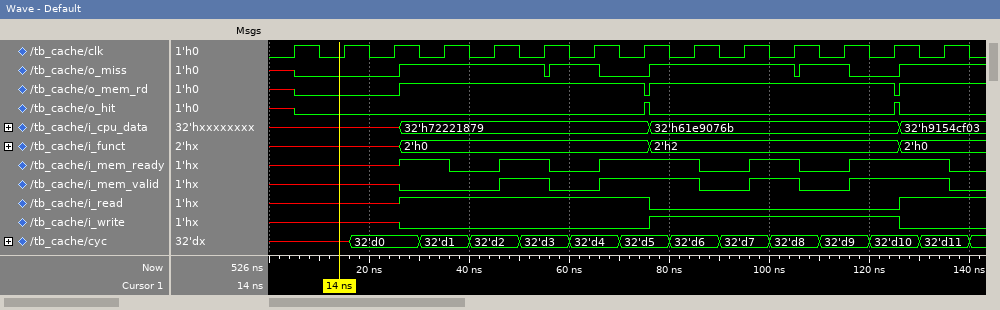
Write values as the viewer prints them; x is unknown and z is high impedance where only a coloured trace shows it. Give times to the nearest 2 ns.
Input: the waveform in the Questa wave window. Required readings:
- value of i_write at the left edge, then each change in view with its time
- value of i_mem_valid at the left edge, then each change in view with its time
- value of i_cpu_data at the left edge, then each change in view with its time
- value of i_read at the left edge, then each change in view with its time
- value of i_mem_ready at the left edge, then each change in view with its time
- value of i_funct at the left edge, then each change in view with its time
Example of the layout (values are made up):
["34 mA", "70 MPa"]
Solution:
["x, 0 at 26 ns, 1 at 76 ns, 0 at 126 ns", "x, 0 at 26 ns, 1 at 46 ns, 0 at 56 ns, 1 at 66 ns, 0 at 86 ns, 1 at 96 ns, 0 at 106 ns, 1 at 116 ns, 0 at 136 ns", "x, 32'h72221879 at 26 ns, 32'h61e9076b at 76 ns, 32'h9154cf03 at 126 ns", "x, 1 at 26 ns, 0 at 76 ns, 1 at 126 ns", "x, 1 at 26 ns, 0 at 36 ns, 1 at 46 ns, 0 at 56 ns, 1 at 66 ns, 0 at 86 ns, 1 at 96 ns, 0 at 106 ns, 1 at 116 ns, 0 at 136 ns", "x, 2'h0 at 26 ns, 2'h2 at 76 ns, 2'h0 at 126 ns"]
